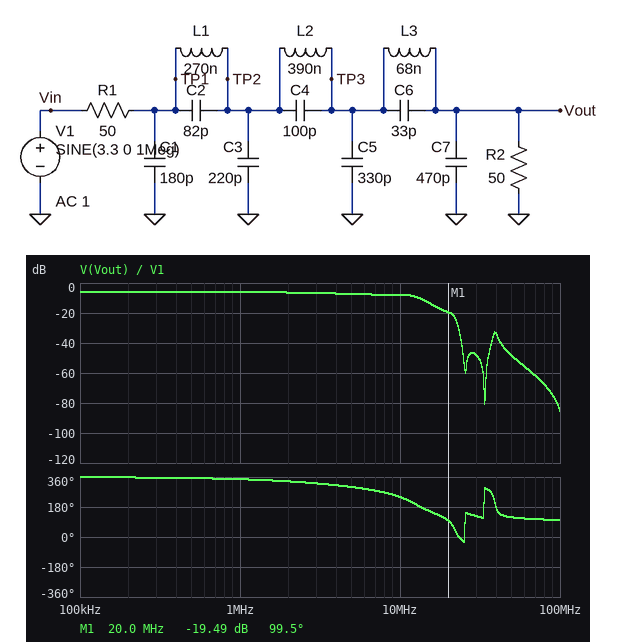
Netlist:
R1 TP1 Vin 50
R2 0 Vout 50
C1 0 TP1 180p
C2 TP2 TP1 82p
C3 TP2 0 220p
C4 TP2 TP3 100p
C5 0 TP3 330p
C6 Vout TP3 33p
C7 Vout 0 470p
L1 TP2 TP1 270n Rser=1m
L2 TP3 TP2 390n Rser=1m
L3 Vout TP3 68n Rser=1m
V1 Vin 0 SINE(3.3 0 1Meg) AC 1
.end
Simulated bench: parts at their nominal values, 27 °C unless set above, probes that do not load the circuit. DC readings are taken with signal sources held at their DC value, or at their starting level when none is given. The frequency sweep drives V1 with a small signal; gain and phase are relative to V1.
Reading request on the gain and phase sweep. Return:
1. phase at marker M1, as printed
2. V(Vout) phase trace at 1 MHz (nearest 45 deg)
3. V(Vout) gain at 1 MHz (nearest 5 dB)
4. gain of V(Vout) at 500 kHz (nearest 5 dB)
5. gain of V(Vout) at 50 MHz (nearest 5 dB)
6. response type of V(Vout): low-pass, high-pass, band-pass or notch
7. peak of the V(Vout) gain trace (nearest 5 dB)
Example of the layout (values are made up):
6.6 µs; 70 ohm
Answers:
99.5 deg; 360 deg; -5 dB; -5 dB; -50 dB; low-pass; -5 dB
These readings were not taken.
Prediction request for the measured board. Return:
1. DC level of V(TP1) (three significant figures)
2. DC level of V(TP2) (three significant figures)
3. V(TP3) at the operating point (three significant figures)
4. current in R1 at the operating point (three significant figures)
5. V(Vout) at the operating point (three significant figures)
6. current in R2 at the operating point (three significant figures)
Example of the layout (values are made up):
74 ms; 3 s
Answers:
1.65 V; 1.65 V; 1.65 V; 33.0 mA; 1.65 V; 33.0 mA
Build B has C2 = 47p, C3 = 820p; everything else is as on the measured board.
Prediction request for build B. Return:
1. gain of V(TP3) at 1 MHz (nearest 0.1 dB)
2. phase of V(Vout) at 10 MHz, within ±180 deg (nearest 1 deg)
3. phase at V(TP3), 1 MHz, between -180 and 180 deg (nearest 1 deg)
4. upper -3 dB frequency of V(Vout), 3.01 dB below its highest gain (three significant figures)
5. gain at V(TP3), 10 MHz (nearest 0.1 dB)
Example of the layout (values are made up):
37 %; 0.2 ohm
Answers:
-6.3 dB; -152 deg; -18 deg; 12.0 MHz; -7.2 dB
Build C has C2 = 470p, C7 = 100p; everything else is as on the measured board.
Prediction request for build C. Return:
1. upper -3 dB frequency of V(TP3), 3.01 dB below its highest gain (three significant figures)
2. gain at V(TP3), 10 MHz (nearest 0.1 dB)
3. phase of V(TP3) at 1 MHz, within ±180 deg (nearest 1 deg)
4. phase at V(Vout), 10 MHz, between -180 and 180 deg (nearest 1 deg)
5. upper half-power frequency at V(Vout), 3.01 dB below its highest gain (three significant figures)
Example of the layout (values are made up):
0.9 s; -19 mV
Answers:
11.8 MHz; -6.8 dB; -10 deg; -113 deg; 11.9 MHz
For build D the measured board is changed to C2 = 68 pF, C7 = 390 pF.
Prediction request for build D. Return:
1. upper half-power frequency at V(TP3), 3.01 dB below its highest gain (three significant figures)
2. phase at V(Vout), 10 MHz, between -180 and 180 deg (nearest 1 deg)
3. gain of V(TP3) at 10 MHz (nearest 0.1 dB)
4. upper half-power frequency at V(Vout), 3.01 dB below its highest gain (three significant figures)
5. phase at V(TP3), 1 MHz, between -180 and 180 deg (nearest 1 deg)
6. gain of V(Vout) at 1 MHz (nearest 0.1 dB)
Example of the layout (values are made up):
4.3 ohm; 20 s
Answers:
11.6 MHz; -116 deg; -8.3 dB; 13.0 MHz; -12 deg; -6.1 dB
